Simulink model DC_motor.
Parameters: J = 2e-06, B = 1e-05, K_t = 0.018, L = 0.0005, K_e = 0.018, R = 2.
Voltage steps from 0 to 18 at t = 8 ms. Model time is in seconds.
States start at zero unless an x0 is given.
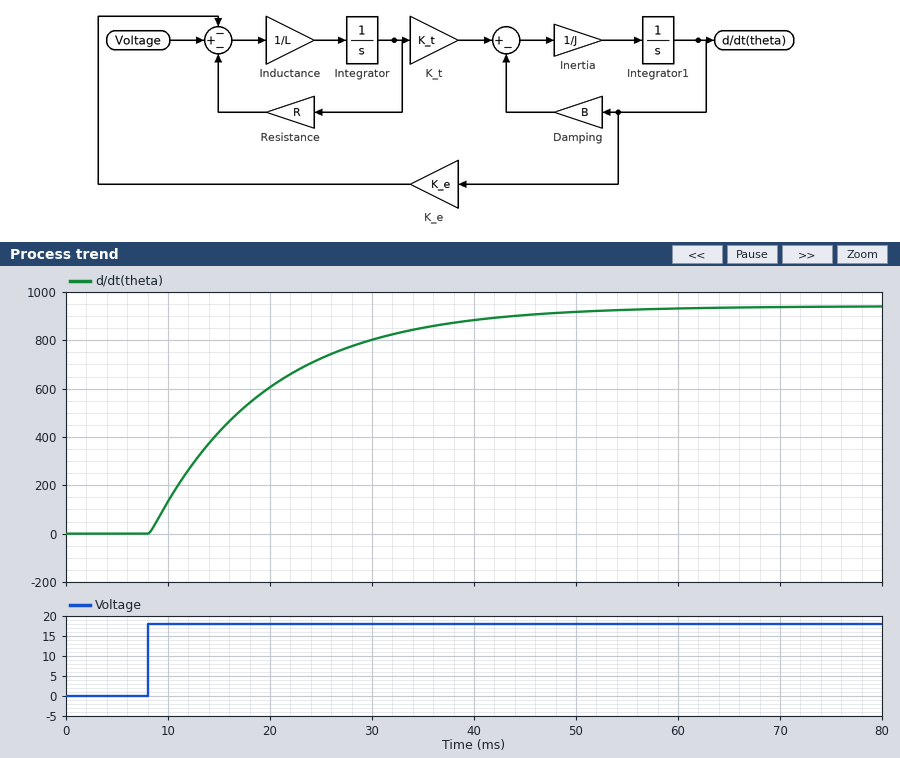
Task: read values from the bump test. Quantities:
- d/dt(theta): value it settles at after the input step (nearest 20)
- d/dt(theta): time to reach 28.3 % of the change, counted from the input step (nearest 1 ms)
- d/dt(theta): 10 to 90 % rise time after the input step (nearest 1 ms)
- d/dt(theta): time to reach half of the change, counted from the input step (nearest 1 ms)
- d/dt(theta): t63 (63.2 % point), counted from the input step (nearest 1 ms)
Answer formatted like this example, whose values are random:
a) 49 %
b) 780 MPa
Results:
a) 940
b) 4 ms
c) 25 ms
d) 8 ms
e) 12 ms
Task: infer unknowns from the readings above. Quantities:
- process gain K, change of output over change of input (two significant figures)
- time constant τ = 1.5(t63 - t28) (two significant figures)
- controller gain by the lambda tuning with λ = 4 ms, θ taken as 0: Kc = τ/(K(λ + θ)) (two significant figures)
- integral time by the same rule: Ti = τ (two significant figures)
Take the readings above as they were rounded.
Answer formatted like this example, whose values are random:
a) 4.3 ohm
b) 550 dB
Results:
a) 52
b) 12 ms
c) 0.058
d) 12 ms
